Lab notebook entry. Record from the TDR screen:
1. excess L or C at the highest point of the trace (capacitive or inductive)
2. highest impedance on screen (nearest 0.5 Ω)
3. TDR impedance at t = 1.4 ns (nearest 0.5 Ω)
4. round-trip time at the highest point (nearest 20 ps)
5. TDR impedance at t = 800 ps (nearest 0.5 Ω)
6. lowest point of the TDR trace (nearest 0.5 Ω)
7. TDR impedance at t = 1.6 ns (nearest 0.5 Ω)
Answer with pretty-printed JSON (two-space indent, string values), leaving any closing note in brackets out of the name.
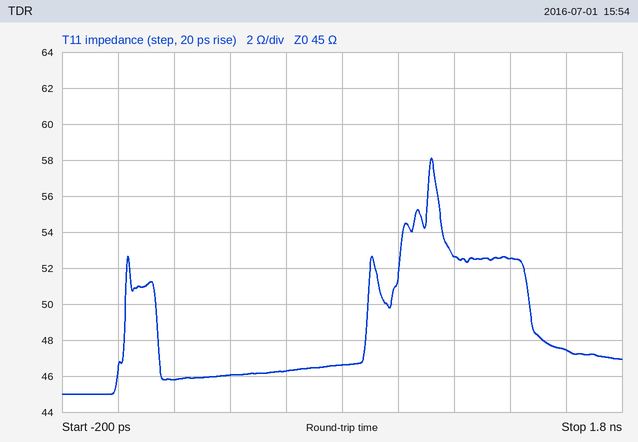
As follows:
{
  "excess L or C at the highest point of the trace": "inductive",
  "highest impedance on screen": "58.0 Ω",
  "TDR impedance at t = 1.4 ns": "52.5 Ω",
  "round-trip time at the highest point": "1.12 ns",
  "TDR impedance at t = 800 ps": "46.5 Ω",
  "lowest point of the TDR trace": "45.0 Ω",
  "TDR impedance at t = 1.6 ns": "47.5 Ω"
}
